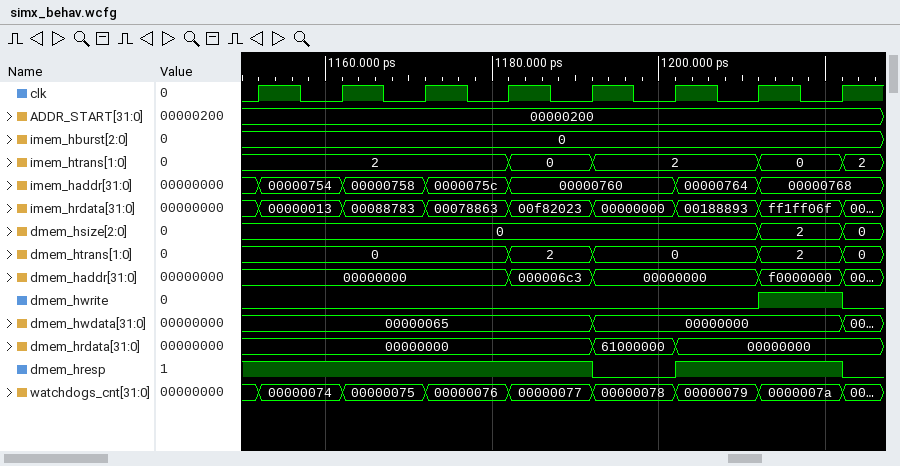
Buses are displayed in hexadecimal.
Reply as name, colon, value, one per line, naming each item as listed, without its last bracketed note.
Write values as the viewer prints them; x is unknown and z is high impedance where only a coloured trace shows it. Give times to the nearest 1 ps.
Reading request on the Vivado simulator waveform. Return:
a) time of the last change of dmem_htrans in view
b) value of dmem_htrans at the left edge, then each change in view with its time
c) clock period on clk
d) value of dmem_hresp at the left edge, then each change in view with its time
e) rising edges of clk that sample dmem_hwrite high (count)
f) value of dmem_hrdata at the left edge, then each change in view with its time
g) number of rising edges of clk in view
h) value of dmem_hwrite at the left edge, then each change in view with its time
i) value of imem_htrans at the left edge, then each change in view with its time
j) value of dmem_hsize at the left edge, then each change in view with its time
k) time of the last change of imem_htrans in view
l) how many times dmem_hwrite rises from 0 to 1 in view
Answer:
time of the last change of dmem_htrans in view: 1222 ps
value of dmem_htrans at the left edge, then each change in view with its time: 0, 2 at 1182 ps, 0 at 1192 ps, 2 at 1212 ps, 0 at 1222 ps
clock period on clk: 10 ps
value of dmem_hresp at the left edge, then each change in view with its time: 1, 0 at 1192 ps, 1 at 1202 ps, 0 at 1222 ps
rising edges of clk that sample dmem_hwrite high: 1
value of dmem_hrdata at the left edge, then each change in view with its time: 00000000, 61000000 at 1192 ps, 00000000 at 1202 ps
number of rising edges of clk in view: 8
value of dmem_hwrite at the left edge, then each change in view with its time: 0, 1 at 1212 ps, 0 at 1222 ps
value of imem_htrans at the left edge, then each change in view with its time: 2, 0 at 1182 ps, 2 at 1192 ps, 0 at 1212 ps, 2 at 1222 ps
value of dmem_hsize at the left edge, then each change in view with its time: 0, 2 at 1212 ps, 0 at 1222 ps
time of the last change of imem_htrans in view: 1222 ps
how many times dmem_hwrite rises from 0 to 1 in view: 1
